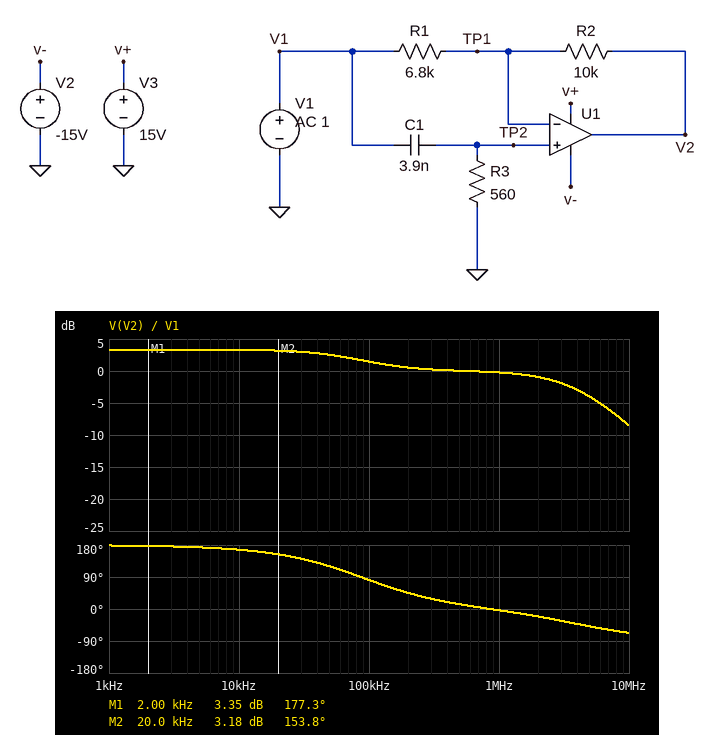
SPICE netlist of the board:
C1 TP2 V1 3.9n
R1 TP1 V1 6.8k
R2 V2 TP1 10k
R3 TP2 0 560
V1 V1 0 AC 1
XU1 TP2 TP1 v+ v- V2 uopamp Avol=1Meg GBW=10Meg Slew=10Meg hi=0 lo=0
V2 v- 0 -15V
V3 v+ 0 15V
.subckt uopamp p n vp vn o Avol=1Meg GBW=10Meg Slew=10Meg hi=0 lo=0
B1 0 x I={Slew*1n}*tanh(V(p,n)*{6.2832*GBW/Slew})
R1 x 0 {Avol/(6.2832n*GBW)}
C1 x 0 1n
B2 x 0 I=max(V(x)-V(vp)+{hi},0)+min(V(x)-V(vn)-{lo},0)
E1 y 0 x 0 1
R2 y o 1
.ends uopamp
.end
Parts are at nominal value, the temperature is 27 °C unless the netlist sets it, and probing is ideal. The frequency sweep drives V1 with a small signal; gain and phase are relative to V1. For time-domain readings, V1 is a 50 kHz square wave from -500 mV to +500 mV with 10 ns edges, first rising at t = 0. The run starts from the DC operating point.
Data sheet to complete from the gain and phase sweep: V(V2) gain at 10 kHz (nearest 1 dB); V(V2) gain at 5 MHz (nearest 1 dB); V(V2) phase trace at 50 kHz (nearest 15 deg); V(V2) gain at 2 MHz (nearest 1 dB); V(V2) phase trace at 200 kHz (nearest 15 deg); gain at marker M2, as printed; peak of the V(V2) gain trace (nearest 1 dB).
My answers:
3 dB
-4 dB
120 deg
-1 dB
45 deg
3.18 dB
3 dB
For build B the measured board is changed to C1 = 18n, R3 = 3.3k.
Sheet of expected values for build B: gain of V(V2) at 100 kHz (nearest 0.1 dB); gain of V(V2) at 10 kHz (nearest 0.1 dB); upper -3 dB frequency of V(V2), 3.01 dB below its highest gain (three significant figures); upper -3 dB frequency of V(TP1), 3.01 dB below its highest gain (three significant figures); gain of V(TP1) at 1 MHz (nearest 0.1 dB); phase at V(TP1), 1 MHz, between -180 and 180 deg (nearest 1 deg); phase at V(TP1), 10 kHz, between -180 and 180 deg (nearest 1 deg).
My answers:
0 dB
0.3 dB
9.77 kHz
7.51 MHz
-0.2 dB
-5 deg
15 deg
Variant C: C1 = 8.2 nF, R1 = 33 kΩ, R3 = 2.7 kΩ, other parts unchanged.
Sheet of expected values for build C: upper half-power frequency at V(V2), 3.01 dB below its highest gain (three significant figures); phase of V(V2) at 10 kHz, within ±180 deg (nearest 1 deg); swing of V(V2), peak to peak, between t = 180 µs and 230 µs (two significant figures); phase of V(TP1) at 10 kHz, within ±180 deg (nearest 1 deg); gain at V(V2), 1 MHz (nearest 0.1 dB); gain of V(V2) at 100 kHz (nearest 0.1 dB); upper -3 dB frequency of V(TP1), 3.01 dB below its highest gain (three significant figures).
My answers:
7.69 MHz
48 deg
1.3 V
36 deg
-0.1 dB
0 dB
8.14 MHz
